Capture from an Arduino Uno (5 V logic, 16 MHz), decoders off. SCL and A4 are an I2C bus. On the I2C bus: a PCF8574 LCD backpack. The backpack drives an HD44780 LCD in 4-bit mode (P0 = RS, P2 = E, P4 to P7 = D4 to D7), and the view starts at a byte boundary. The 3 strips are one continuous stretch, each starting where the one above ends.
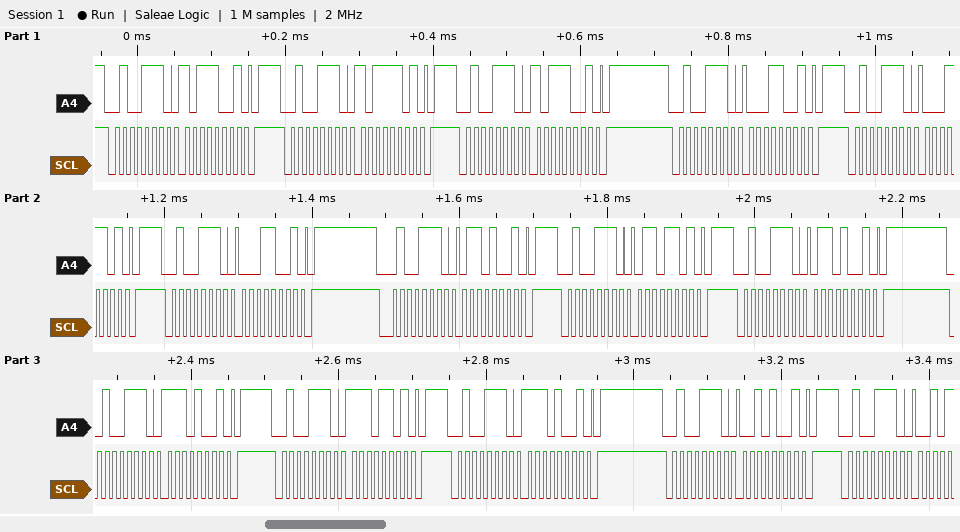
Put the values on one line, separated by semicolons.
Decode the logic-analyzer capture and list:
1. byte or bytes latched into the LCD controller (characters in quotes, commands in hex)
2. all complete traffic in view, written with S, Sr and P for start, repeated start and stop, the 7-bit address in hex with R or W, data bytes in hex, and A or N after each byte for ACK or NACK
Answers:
data 0xB1 'n'; S 27W A B9 A P S 27W A BD A P S 27W A B9 A P S 27W A 19 A P S 27W A 1D A P S 27W A 19 A P S 27W A 69 A P S 27W A 6D A P S 27W A 69 A P S 27W A E9 A P S 27W A ED A P S 27W A E9 A P S 27W A 29 A P S 27W A
